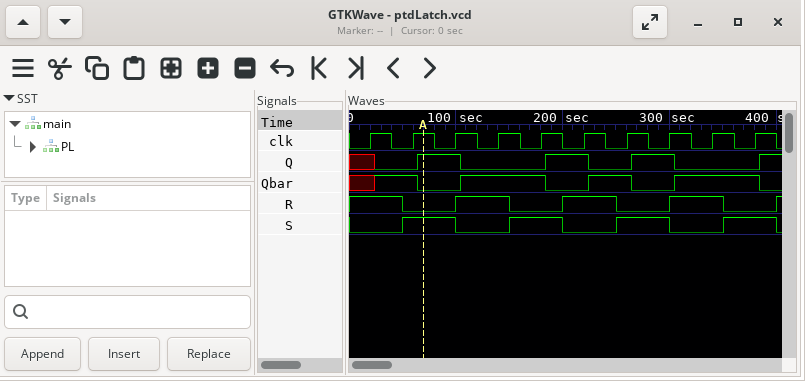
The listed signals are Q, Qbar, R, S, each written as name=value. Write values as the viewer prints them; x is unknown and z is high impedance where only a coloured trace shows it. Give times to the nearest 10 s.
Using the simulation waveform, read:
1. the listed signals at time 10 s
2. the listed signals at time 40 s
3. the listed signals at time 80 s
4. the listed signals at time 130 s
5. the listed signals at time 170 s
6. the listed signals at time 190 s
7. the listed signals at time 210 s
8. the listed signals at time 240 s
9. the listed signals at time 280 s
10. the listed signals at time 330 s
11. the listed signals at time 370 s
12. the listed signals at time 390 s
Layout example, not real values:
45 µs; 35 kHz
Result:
Q=x, Qbar=x, R=1, S=0; Q=0, Qbar=1, R=1, S=0; Q=1, Qbar=0, R=0, S=1; Q=0, Qbar=1, R=1, S=0; Q=0, Qbar=1, R=0, S=1; Q=1, Qbar=0, R=0, S=1; Q=1, Qbar=0, R=1, S=0; Q=0, Qbar=1, R=1, S=0; Q=1, Qbar=0, R=0, S=1; Q=0, Qbar=1, R=1, S=0; Q=0, Qbar=1, R=0, S=1; Q=1, Qbar=0, R=0, S=1
